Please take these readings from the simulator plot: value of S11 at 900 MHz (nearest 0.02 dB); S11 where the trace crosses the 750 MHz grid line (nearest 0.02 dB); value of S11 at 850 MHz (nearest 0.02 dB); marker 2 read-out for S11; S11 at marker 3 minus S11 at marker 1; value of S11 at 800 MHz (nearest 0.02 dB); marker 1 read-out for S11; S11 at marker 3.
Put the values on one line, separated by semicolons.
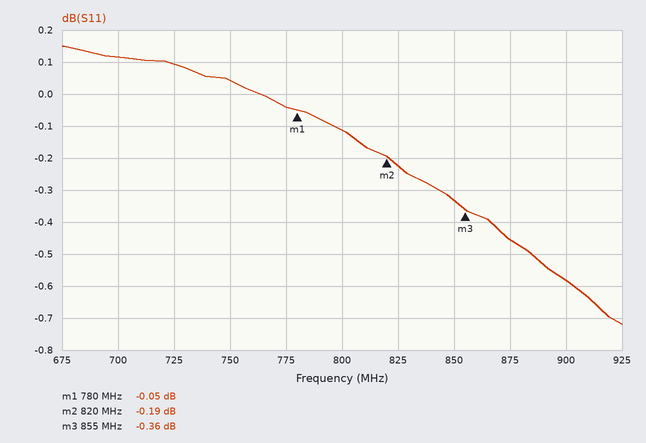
-0.58 dB; 0.04 dB; -0.34 dB; -0.19 dB; -0.31 dB; -0.12 dB; -0.05 dB; -0.36 dB
